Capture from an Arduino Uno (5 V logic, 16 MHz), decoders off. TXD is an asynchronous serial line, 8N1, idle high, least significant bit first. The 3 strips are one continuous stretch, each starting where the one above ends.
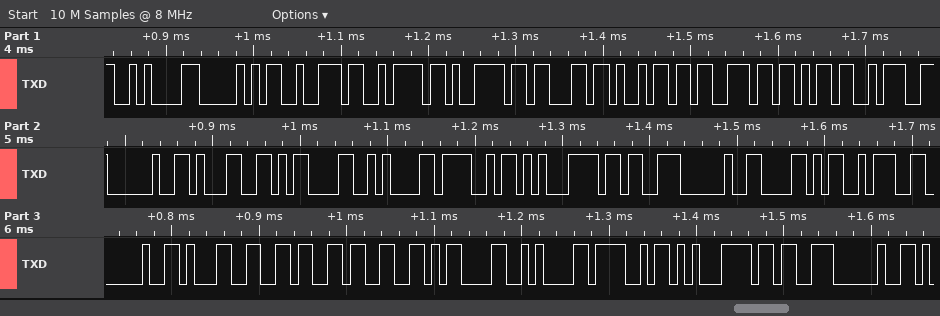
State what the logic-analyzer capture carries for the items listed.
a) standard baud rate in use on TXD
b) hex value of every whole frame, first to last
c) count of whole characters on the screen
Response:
115200 baud
0x0A 0x50 0x72 0x7A 0x79 0x63 0x69 0x73 0x6B 0x3A 0x20 0x31 0x0D 0x0A 0x4F 0xC5 0x9B 0x20 0x58 0x3A 0x20 0x31 0x36 0x33 0x0D 0x0A 0x4F 0xC5 0x9B 0x20
30
